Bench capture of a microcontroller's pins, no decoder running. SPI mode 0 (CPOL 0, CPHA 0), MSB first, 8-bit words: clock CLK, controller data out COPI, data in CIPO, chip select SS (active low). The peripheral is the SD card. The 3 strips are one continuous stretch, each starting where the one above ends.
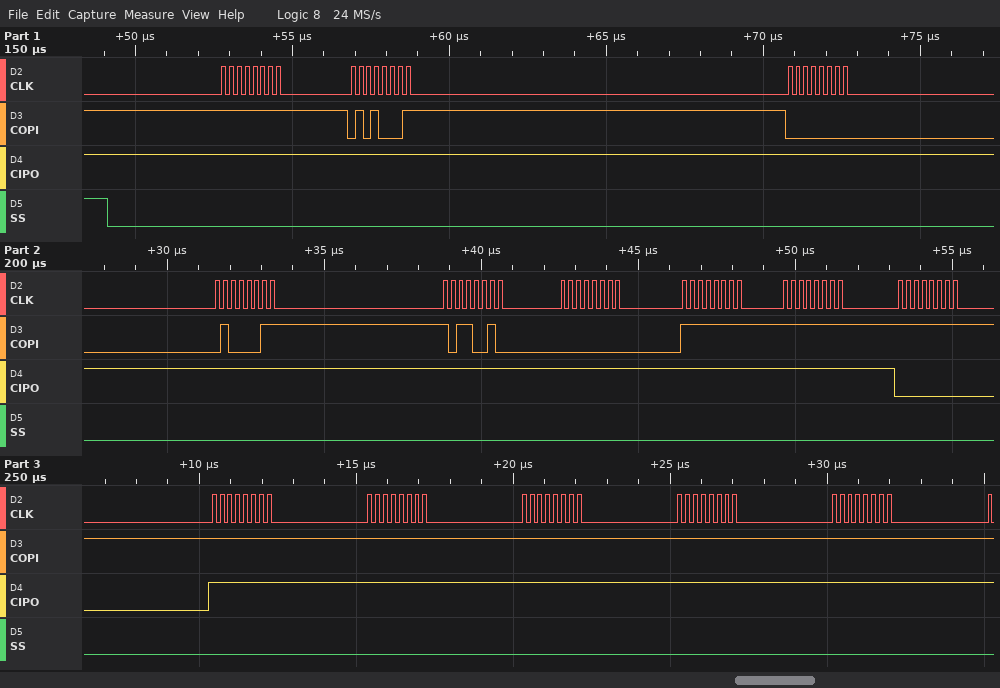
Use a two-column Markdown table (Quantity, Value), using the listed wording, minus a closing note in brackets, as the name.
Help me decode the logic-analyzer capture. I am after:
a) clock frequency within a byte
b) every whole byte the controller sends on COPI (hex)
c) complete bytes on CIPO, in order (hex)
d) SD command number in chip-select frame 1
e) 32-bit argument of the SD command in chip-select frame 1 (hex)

| Quantity | Value |
|---|---|
| clock frequency within a byte | 4 MHz |
| every whole byte the controller sends on COPI | FF 51 00 43 B2 00 FF FF FF FF FF FF FF FF |
| complete bytes on CIPO, in order | FF FF FF FF FF FF FF FF 00 FF FF FF FF FF |
| SD command number in chip-select frame 1 | CMD17 |
| 32-bit argument of the SD command in chip-select frame 1 | 0x0043B200 |
